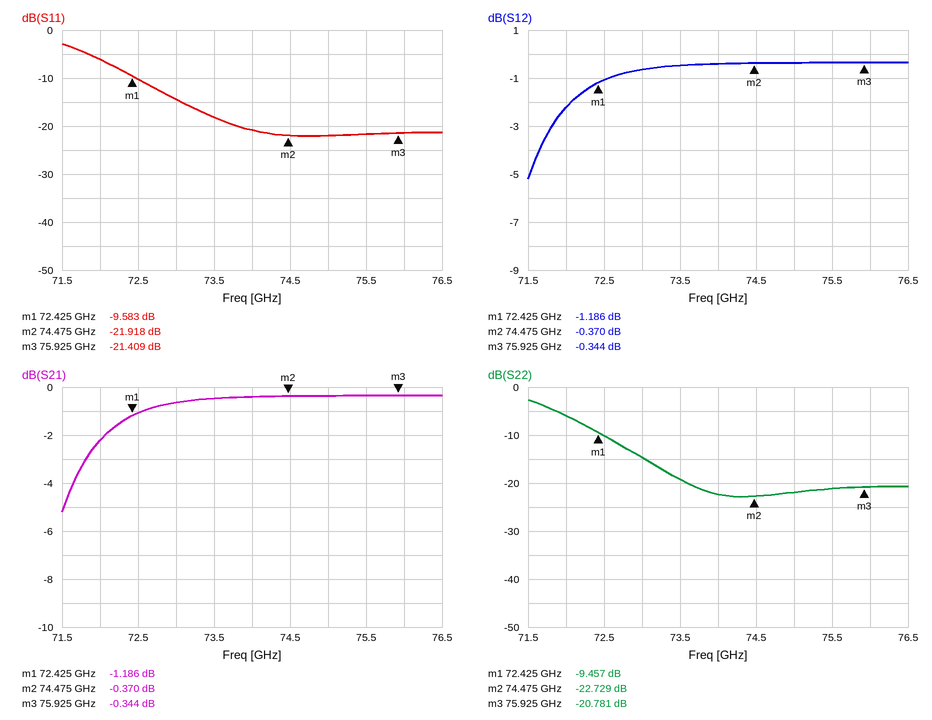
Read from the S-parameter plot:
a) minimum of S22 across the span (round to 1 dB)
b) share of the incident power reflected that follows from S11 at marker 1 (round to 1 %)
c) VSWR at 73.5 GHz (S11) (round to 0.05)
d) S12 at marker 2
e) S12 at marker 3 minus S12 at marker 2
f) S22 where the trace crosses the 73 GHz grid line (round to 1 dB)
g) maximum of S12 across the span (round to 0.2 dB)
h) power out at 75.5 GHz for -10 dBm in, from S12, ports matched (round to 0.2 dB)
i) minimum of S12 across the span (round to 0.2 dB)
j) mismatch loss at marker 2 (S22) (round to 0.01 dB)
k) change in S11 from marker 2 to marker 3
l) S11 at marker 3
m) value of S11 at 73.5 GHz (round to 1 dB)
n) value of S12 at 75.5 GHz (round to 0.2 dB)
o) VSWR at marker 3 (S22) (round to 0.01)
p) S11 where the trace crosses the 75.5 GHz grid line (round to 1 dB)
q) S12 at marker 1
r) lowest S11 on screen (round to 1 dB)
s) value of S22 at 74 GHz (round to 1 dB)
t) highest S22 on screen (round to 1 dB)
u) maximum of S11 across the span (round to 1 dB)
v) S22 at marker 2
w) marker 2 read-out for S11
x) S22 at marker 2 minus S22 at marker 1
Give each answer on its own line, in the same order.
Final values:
-23 dB
11 %
1.30
-0.370 dB
0.026 dB
-15 dB
-0.4 dB
-10.4 dBm
-5.2 dB
0.02 dB
0.509 dB
-21.409 dB
-18 dB
-0.4 dB
1.20
-22 dB
-1.186 dB
-22 dB
-22 dB
-3 dB
-3 dB
-22.729 dB
-21.918 dB
-13.272 dB
